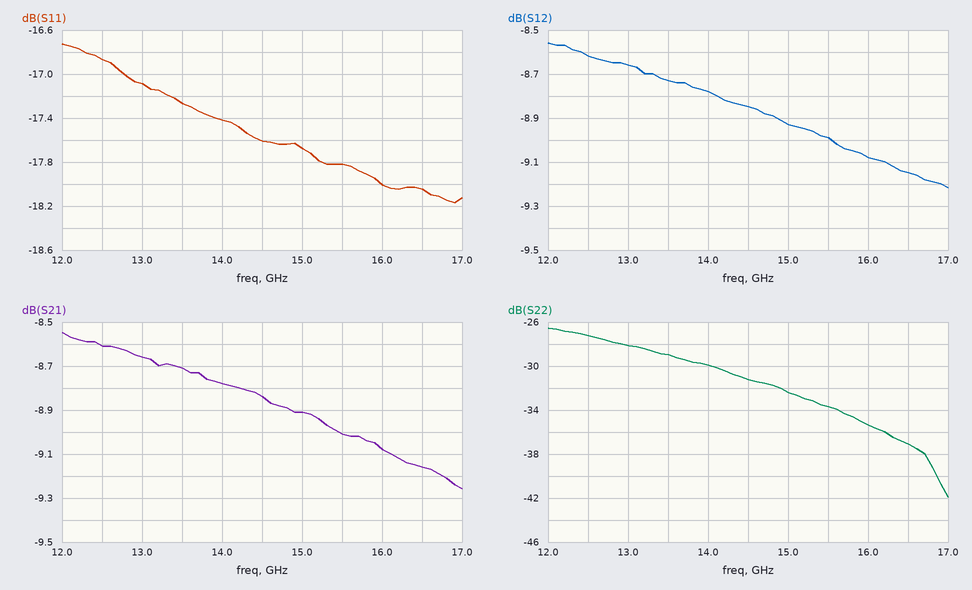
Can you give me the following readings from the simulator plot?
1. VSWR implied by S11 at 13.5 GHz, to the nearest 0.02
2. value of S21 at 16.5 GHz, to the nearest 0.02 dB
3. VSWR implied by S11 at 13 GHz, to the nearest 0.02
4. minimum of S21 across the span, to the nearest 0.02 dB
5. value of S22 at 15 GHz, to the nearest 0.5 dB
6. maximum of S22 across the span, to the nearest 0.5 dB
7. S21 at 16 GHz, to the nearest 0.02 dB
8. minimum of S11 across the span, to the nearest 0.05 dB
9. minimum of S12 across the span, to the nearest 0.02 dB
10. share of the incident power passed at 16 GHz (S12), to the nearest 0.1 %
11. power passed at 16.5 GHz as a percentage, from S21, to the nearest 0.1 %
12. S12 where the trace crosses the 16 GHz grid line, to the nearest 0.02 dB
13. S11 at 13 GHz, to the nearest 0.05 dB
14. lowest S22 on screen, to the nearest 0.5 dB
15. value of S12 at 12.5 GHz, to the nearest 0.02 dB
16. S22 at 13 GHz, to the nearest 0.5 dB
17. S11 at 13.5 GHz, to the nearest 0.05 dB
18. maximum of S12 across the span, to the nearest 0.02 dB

1.32
-9.16 dB
1.32
-9.26 dB
-32.5 dB
-26.5 dB
-9.08 dB
-18.15 dB
-9.22 dB
12.4 %
12.1 %
-9.08 dB
-17.10 dB
-42.0 dB
-8.62 dB
-28.0 dB
-17.25 dB
-8.56 dB
